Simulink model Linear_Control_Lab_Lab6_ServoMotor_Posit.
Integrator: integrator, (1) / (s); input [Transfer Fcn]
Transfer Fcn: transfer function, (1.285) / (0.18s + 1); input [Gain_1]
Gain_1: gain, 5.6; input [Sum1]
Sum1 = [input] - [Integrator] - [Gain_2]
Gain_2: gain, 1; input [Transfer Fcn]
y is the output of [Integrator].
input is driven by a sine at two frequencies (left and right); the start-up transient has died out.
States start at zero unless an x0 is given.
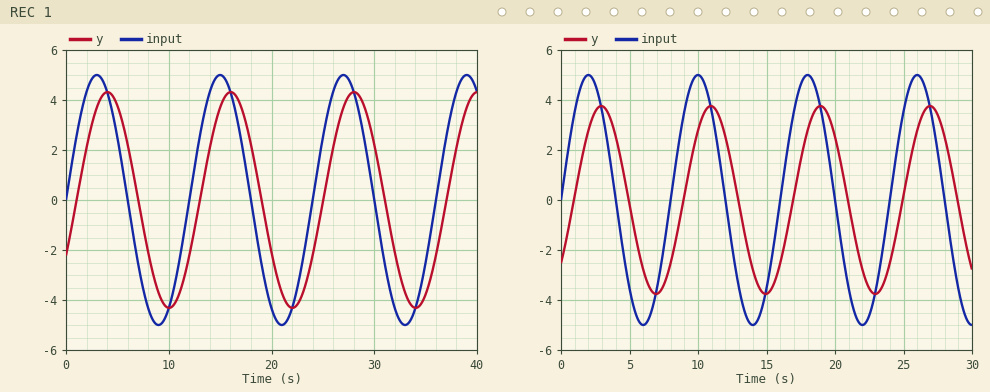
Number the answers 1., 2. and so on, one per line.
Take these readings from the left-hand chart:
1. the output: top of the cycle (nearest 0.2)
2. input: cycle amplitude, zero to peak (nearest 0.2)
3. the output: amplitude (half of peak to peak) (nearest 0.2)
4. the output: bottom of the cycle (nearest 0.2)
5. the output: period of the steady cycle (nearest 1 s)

1. 4.4
2. 5.0
3. 4.4
4. -4.4
5. 12 s
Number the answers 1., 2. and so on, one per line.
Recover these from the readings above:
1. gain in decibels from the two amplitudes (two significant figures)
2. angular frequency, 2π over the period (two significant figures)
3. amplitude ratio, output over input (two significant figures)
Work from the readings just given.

1. -1.1 dB
2. 0.52 rad/s
3. 0.88
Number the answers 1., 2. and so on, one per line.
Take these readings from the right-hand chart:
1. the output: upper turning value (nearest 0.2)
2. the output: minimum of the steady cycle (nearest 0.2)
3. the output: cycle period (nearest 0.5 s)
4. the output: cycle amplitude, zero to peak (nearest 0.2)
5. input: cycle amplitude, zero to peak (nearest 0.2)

1. 3.8
2. -3.8
3. 8.0 s
4. 3.8
5. 5.0
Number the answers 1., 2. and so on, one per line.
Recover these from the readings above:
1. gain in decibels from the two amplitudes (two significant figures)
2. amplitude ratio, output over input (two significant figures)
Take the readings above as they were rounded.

1. -2.4 dB
2. 0.76
